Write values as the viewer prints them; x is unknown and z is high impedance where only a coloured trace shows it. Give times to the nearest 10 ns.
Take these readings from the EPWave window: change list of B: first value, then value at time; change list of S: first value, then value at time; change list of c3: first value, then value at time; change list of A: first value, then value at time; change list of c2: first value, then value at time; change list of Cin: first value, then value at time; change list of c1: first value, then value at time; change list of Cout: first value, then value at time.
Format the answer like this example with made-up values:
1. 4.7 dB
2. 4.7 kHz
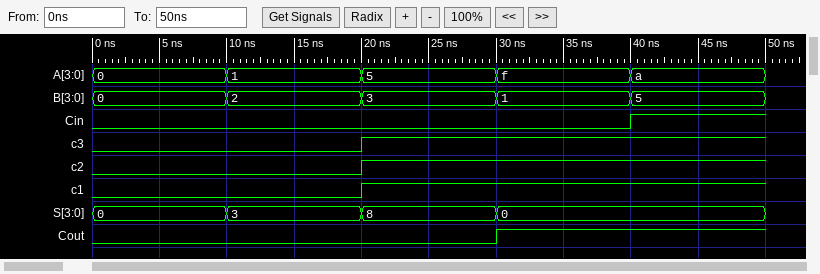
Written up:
1. 0, 2 at 10 ns, 3 at 20 ns, 1 at 30 ns, 5 at 40 ns
2. 0, 3 at 10 ns, 8 at 20 ns, 0 at 30 ns
3. 0, 1 at 20 ns
4. 0, 1 at 10 ns, 5 at 20 ns, f at 30 ns, a at 40 ns
5. 0, 1 at 20 ns
6. 0, 1 at 40 ns
7. 0, 1 at 20 ns
8. 0, 1 at 30 ns
